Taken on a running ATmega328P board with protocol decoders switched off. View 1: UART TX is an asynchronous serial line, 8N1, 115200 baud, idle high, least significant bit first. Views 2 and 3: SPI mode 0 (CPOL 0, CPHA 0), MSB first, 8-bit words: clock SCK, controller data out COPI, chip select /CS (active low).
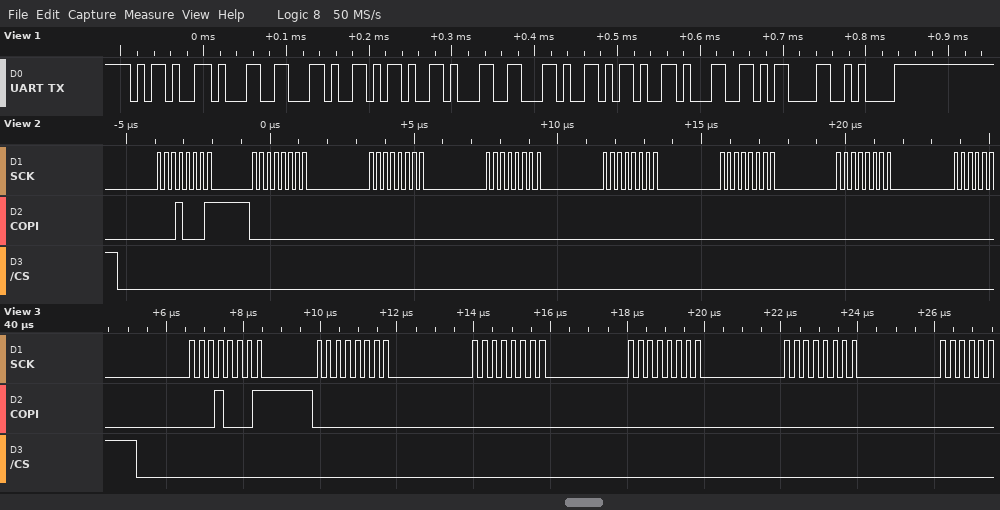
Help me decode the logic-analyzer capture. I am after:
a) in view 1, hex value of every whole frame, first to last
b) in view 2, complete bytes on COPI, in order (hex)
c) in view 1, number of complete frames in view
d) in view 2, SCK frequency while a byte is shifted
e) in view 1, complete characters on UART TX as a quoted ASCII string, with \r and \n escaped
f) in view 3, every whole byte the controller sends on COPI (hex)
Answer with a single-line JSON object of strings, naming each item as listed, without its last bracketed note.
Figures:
{"in view 1, hex value of every whole frame, first to last": "0x2D 0x31 0x2C 0x2D 0x31 0x2C 0x2D 0x31 0x0D 0x0A", "in view 2, complete bytes on COPI, in order": "0x11 0x00 0x00 0x00 0x00 0x00 0x00", "in view 1, number of complete frames in view": "10", "in view 2, SCK frequency while a byte is shifted": "4 MHz", "in view 1, complete characters on UART TX as a quoted ASCII string, with \\r and \\n escaped": "\"-1,-1,-1\\r\\n\"", "in view 3, every whole byte the controller sends on COPI": "0x11 0x00 0x00 0x00 0x00"}
